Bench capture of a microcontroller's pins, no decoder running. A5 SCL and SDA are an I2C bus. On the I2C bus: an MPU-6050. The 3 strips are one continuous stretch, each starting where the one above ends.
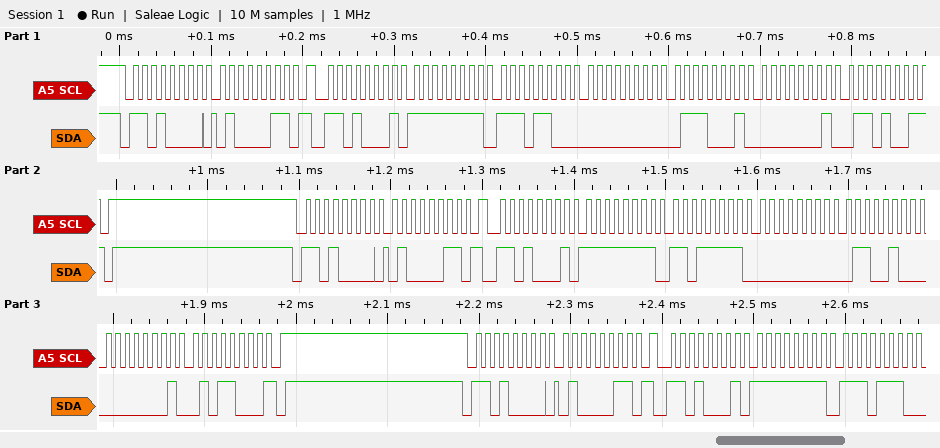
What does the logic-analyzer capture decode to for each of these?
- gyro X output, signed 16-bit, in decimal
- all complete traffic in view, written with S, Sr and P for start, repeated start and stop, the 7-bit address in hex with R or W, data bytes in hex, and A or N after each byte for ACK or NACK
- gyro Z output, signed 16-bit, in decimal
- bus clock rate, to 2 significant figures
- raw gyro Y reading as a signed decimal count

-20
S 68W A 43 A Sr 68R A FF A EC A 00 A 71 A 01 A 69 N P S 68W A 43 A Sr 68R A FF A DF A 00 A 64 A 01 A 58 N P S 68W A 43 A Sr 68R A FF A EE A
361
100 kHz
113
